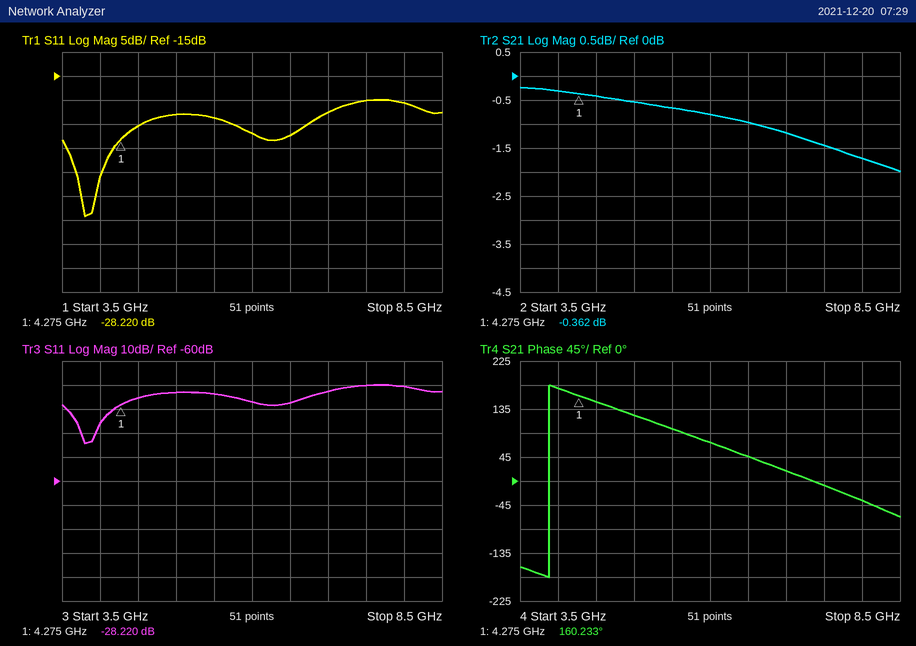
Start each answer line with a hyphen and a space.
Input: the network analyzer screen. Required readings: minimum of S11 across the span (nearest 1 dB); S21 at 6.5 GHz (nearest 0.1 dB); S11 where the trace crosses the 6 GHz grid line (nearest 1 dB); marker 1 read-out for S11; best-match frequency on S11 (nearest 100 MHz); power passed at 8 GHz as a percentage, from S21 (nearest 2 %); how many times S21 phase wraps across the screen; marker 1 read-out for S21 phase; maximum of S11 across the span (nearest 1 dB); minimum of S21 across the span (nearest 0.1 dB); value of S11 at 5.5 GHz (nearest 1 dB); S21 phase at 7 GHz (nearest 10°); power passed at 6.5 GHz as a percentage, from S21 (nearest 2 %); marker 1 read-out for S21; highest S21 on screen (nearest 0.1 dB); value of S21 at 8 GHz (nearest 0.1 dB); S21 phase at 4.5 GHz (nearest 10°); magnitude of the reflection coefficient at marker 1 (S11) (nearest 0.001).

- -44 dB
- -1.0 dB
- -27 dB
- -28.220 dB
- 3.8 GHz
- 68 %
- 1
- 160.233°
- -20 dB
- -2.0 dB
- -24 dB
- 20°
- 80 %
- -0.362 dB
- -0.2 dB
- -1.7 dB
- 150°
- 0.039
